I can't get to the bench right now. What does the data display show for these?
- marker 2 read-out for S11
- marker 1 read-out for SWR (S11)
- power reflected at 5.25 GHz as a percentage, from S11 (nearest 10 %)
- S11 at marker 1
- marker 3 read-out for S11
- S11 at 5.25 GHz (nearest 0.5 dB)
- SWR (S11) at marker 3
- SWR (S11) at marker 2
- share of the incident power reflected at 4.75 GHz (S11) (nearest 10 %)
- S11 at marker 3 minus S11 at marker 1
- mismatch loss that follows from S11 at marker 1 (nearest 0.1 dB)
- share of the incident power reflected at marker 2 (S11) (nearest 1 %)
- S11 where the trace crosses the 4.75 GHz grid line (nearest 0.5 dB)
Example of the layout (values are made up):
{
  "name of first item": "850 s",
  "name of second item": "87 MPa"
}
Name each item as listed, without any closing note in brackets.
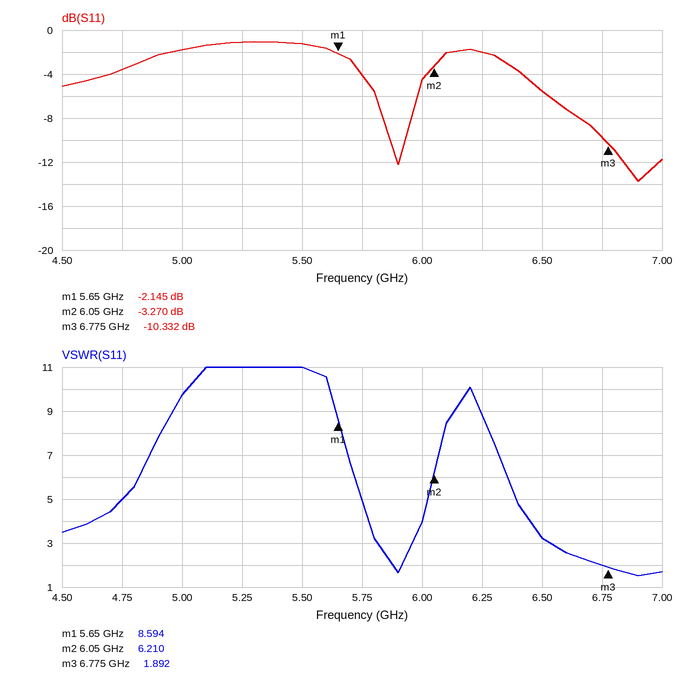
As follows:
{
  "marker 2 read-out for S11": "-3.270 dB",
  "marker 1 read-out for SWR": "8.594",
  "power reflected at 5.25 GHz as a percentage, from S11": "80 %",
  "S11 at marker 1": "-2.145 dB",
  "marker 3 read-out for S11": "-10.332 dB",
  "S11 at 5.25 GHz": "-1.0 dB",
  "SWR (S11) at marker 3": "1.892",
  "SWR (S11) at marker 2": "6.210",
  "share of the incident power reflected at 4.75 GHz (S11)": "40 %",
  "S11 at marker 3 minus S11 at marker 1": "-8.187 dB",
  "mismatch loss that follows from S11 at marker 1": "4.1 dB",
  "share of the incident power reflected at marker 2 (S11)": "47 %",
  "S11 where the trace crosses the 4.75 GHz grid line": "-3.5 dB"
}
